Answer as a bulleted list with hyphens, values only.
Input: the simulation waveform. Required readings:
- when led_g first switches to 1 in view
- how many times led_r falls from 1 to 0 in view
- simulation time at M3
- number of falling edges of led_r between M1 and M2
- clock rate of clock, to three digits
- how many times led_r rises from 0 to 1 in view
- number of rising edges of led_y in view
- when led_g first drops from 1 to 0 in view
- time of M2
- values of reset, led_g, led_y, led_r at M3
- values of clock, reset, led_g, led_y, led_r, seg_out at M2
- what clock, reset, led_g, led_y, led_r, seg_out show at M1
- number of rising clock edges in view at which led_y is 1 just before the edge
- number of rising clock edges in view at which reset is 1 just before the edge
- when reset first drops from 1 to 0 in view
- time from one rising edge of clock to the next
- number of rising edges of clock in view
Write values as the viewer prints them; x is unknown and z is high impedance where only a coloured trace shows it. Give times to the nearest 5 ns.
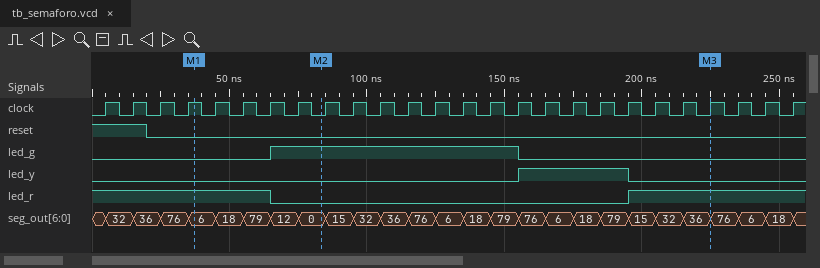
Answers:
- 65 ns
- 1
- 225 ns
- 1
- 100 MHz
- 1
- 1
- 155 ns
- 85 ns
- reset=0, led_g=0, led_y=0, led_r=1
- clock=0, reset=0, led_g=1, led_y=0, led_r=0, seg_out=0
- clock=1, reset=0, led_g=0, led_y=0, led_r=1, seg_out=6
- 4
- 2
- 20 ns
- 10 ns
- 26
